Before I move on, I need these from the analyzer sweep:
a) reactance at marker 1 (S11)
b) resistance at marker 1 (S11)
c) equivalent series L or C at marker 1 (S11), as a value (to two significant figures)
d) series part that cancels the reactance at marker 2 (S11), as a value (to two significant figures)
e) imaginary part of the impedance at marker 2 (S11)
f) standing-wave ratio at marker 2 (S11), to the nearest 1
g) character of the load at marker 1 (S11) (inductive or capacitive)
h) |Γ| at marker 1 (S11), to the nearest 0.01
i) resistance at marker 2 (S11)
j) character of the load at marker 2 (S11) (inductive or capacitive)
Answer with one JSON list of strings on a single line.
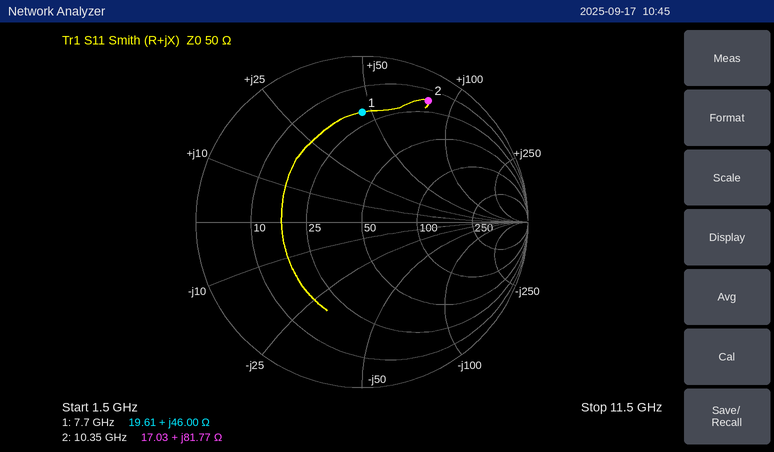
["+46.00 Ω", "19.61 Ω", "950 pH", "190 fF", "+81.77 Ω", "11", "inductive", "0.66", "17.03 Ω", "inductive"]
